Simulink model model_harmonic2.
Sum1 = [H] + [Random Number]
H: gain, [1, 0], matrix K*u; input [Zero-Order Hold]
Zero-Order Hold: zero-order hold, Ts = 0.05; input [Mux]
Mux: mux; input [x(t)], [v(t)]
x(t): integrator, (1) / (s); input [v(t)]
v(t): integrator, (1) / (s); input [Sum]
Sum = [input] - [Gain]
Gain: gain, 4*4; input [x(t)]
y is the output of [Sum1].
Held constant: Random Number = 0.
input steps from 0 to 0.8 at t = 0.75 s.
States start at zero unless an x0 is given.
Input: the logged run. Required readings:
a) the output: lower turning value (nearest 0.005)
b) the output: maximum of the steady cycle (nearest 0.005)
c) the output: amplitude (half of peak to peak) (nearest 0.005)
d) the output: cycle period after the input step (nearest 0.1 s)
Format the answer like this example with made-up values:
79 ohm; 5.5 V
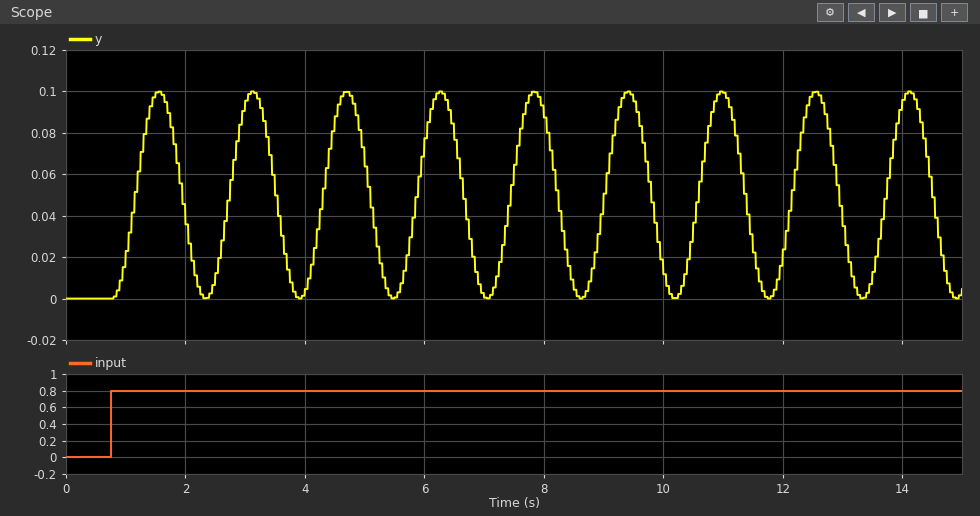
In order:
0.000; 0.100; 0.050; 1.6 s
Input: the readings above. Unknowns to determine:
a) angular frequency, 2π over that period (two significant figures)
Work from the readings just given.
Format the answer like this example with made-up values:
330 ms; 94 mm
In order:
3.9 rad/s
